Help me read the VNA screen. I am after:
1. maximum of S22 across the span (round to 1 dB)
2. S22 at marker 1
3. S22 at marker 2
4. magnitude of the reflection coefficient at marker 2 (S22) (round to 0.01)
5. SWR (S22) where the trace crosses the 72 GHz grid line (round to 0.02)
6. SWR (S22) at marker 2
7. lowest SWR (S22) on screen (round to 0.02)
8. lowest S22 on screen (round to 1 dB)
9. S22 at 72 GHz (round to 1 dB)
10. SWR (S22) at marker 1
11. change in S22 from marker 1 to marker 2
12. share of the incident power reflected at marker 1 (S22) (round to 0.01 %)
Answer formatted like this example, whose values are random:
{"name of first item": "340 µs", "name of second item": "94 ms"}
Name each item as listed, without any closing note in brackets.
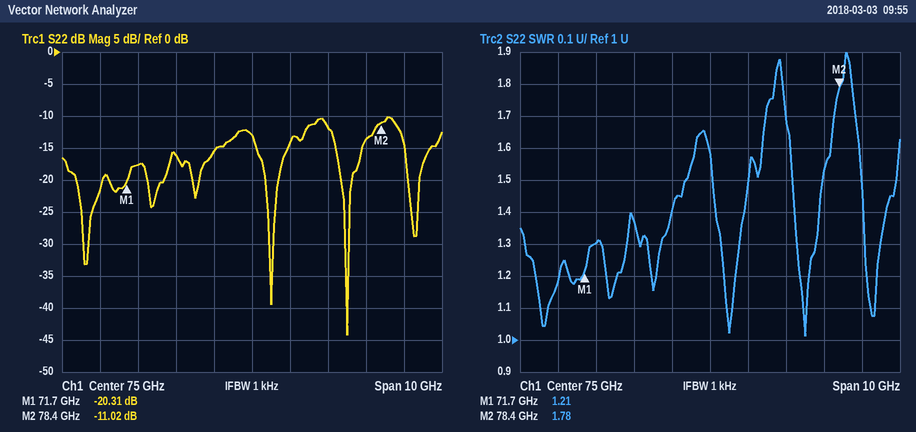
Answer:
{"maximum of S22 across the span": "-10 dB", "S22 at marker 1": "-20.31 dB", "S22 at marker 2": "-11.02 dB", "magnitude of the reflection coefficient at marker 2 (S22)": "0.28", "SWR (S22) where the trace crosses the 72 GHz grid line": "1.30", "SWR (S22) at marker 2": "1.78", "lowest SWR (S22) on screen": "1.02", "lowest S22 on screen": "-44 dB", "S22 at 72 GHz": "-18 dB", "SWR (S22) at marker 1": "1.21", "change in S22 from marker 1 to marker 2": "9.29 dB", "share of the incident power reflected at marker 1 (S22)": "0.93 %"}
